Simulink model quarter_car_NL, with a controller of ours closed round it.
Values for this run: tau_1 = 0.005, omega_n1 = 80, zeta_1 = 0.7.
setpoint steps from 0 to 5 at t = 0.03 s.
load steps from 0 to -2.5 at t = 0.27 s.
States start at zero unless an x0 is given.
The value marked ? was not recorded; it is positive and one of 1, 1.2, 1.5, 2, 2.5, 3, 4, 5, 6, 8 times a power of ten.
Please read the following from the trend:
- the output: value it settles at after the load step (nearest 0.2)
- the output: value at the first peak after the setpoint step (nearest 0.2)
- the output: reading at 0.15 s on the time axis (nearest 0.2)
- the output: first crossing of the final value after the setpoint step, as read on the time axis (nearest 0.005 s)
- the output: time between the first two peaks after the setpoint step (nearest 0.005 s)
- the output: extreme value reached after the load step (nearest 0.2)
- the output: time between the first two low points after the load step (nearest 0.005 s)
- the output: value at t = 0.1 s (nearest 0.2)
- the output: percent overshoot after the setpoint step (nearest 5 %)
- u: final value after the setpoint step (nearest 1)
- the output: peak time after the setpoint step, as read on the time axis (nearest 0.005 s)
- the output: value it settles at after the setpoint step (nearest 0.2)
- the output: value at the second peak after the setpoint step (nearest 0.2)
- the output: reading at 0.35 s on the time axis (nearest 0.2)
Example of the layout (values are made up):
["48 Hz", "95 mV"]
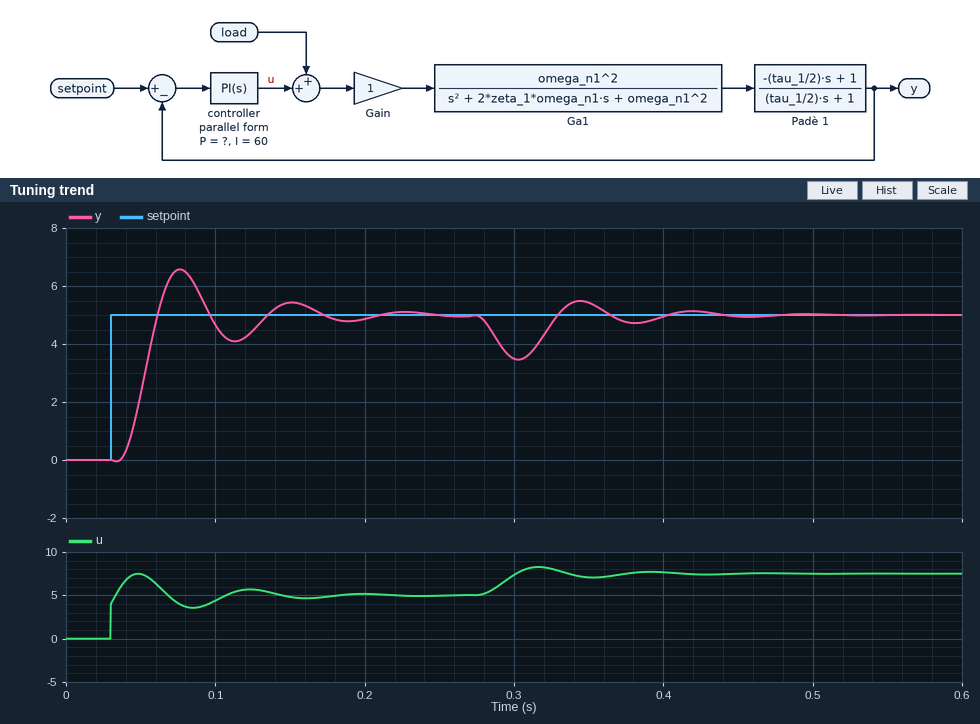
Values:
["5.0", "6.6", "5.4", "0.060 s", "0.075 s", "3.4", "0.080 s", "4.6", "30 %", "5", "0.075 s", "5.0", "5.4", "5.4"]
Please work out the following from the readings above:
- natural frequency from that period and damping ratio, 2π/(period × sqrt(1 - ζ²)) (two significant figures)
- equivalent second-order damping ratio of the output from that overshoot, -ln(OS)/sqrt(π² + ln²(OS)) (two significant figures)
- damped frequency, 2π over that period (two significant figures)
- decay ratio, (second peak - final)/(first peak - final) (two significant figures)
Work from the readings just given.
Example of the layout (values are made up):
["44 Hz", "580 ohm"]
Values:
["90 rad/s", "0.36", "84 rad/s", "0.25"]
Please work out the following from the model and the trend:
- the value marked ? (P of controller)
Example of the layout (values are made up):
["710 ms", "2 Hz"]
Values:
["0.8"]
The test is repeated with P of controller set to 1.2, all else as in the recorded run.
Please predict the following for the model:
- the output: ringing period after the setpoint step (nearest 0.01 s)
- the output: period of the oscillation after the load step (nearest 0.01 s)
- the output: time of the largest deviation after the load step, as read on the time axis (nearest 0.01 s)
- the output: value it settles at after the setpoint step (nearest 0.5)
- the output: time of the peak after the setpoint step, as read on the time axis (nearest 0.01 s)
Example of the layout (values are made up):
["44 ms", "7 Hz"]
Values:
["0.06 s", "0.07 s", "0.30 s", "5.0", "0.07 s"]
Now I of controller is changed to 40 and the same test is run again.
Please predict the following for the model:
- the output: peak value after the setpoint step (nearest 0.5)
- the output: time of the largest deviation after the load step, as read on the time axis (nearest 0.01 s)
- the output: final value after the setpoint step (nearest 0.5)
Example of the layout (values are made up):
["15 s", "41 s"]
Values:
["5.5", "0.30 s", "5.0"]
